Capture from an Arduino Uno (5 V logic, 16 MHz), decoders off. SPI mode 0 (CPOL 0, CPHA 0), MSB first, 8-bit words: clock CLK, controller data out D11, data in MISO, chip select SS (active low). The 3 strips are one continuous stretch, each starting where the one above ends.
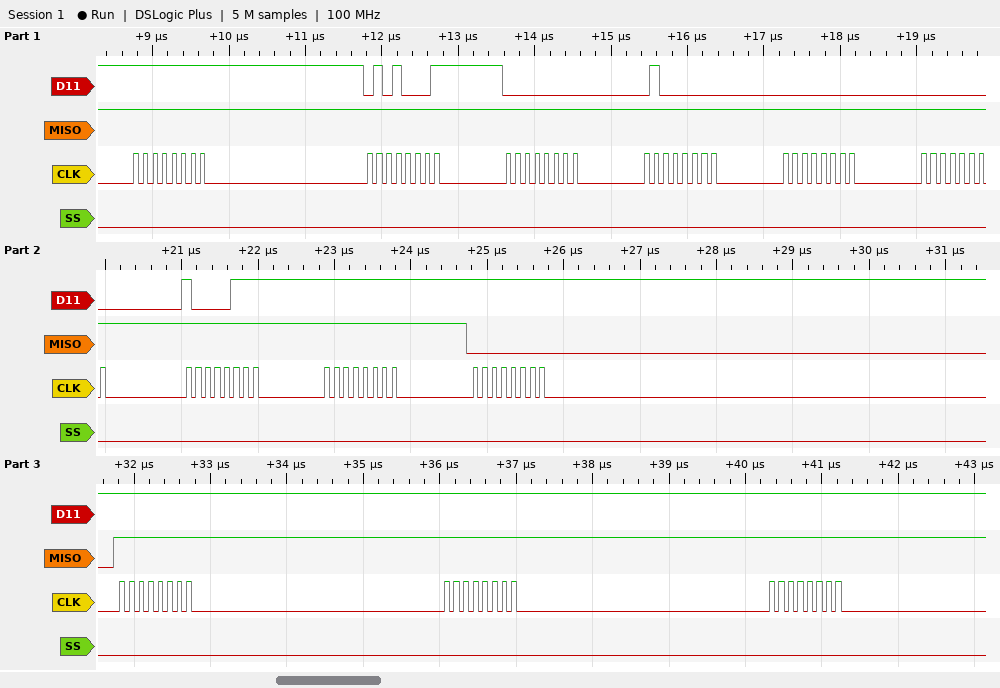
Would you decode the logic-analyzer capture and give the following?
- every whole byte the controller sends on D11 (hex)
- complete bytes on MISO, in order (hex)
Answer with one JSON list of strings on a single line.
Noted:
["FF 51 00 40 00 00 87 FF FF FF FF FF", "FF FF FF FF FF FF FF FF 00 FF FF FF"]
